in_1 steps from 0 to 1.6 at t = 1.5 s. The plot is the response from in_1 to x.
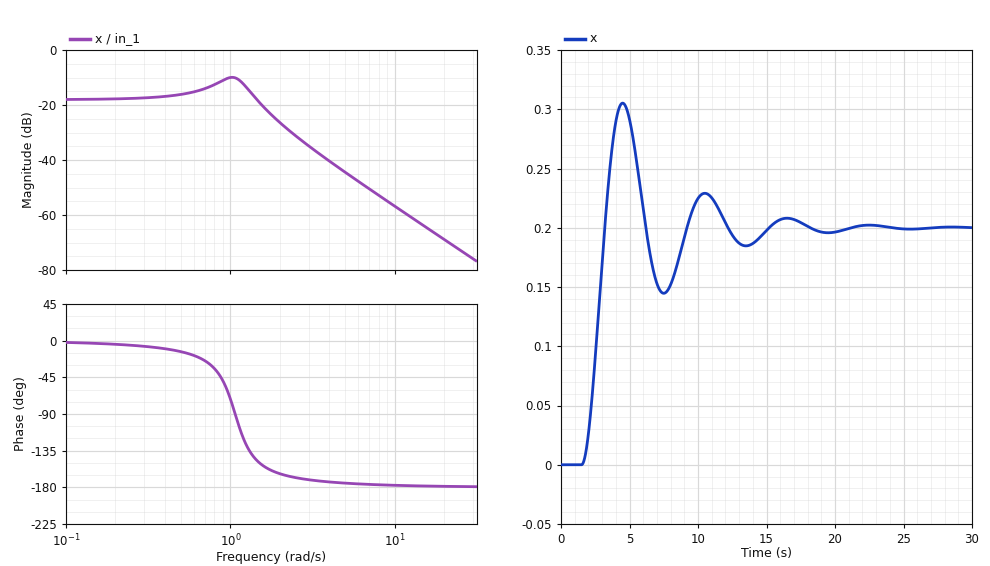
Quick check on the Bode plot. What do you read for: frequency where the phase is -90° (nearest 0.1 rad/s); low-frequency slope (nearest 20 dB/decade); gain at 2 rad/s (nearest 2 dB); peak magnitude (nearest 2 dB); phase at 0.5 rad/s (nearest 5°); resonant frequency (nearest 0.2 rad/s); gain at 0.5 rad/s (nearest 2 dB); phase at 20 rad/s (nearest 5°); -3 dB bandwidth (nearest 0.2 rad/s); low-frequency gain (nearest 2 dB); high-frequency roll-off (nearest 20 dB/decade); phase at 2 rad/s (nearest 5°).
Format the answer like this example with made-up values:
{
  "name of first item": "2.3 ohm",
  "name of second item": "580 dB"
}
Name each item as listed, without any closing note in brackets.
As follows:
{
  "frequency where the phase is -90°": "1.1 rad/s",
  "low-frequency slope": "0 dB/decade",
  "gain at 2 rad/s": "-26 dB",
  "peak magnitude": "-10 dB",
  "phase at 0.5 rad/s": "-15°",
  "resonant frequency": "1.0 rad/s",
  "gain at 0.5 rad/s": "-16 dB",
  "phase at 20 rad/s": "-180°",
  "-3 dB bandwidth": "1.6 rad/s",
  "low-frequency gain": "-18 dB",
  "high-frequency roll-off": "-40 dB/decade",
  "phase at 2 rad/s": "-165°"
}
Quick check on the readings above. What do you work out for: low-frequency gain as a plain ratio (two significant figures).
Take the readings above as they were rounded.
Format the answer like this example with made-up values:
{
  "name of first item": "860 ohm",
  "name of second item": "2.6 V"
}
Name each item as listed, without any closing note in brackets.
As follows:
{
  "low-frequency gain as a plain ratio": "0.13"
}
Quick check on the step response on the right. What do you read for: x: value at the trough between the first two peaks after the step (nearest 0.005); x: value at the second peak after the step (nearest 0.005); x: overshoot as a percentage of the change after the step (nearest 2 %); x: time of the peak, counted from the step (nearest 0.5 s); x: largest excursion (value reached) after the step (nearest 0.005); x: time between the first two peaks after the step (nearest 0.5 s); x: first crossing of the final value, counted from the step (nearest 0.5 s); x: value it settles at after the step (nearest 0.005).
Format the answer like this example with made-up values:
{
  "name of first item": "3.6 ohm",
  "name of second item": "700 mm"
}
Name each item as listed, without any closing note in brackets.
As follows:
{
  "x: value at the trough between the first two peaks after the step": "0.145",
  "x: value at the second peak after the step": "0.230",
  "x: overshoot as a percentage of the change after the step": "52 %",
  "x: time of the peak, counted from the step": "3.0 s",
  "x: largest excursion (value reached) after the step": "0.305",
  "x: time between the first two peaks after the step": "6.0 s",
  "x: first crossing of the final value, counted from the step": "1.5 s",
  "x: value it settles at after the step": "0.200"
}
